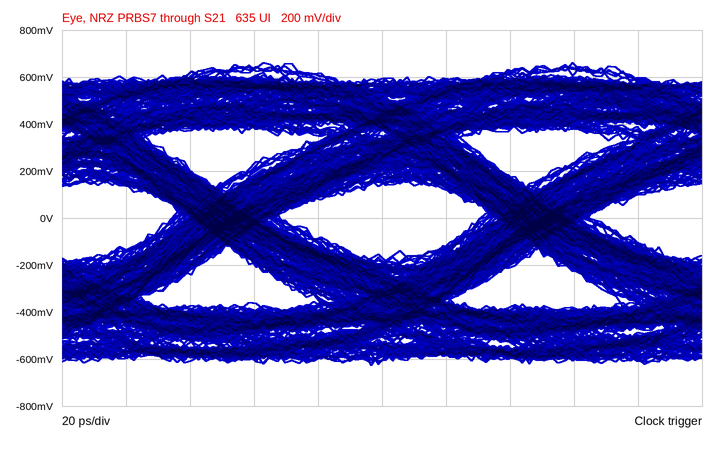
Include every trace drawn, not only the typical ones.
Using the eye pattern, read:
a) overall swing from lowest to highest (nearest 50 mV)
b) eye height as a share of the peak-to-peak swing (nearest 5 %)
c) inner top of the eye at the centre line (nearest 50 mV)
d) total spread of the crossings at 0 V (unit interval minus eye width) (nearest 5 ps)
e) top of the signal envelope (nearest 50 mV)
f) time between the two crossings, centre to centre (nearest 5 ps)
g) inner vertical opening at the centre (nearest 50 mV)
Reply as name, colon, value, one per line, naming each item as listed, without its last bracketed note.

overall swing from lowest to highest: 1.30 V
eye height as a share of the peak-to-peak swing: 25 %
inner top of the eye at the centre line: 150 mV
total spread of the crossings at 0 V (unit interval minus eye width): 35 ps
top of the signal envelope: 650 mV
time between the two crossings, centre to centre: 95 ps
inner vertical opening at the centre: 300 mV
